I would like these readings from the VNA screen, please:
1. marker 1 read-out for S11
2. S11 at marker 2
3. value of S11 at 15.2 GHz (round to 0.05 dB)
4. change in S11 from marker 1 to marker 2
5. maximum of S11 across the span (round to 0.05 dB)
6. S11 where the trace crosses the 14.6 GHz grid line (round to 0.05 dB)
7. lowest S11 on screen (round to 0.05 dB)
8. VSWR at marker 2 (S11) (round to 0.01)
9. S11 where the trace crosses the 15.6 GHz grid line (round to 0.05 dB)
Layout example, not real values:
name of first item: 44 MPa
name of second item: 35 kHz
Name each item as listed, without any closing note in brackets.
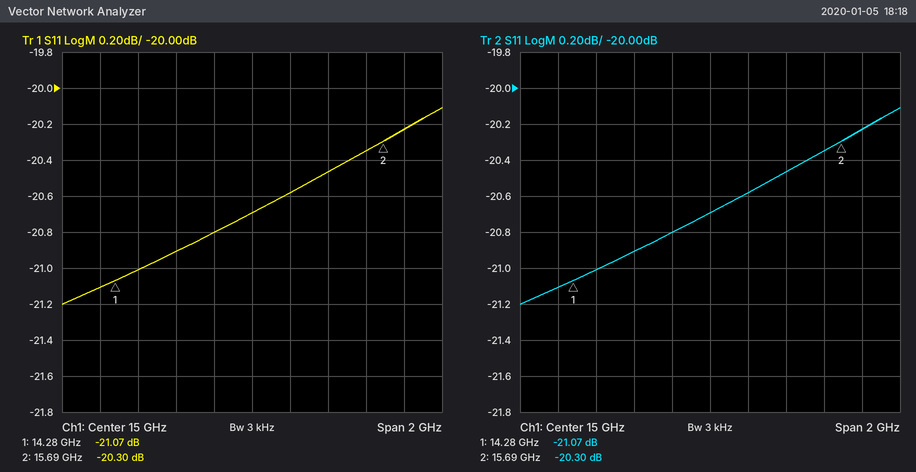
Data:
marker 1 read-out for S11: -21.07 dB
S11 at marker 2: -20.30 dB
value of S11 at 15.2 GHz: -20.60 dB
change in S11 from marker 1 to marker 2: 0.77 dB
maximum of S11 across the span: -20.10 dB
S11 where the trace crosses the 14.6 GHz grid line: -20.90 dB
lowest S11 on screen: -21.20 dB
VSWR at marker 2 (S11): 1.21
S11 where the trace crosses the 15.6 GHz grid line: -20.35 dB
